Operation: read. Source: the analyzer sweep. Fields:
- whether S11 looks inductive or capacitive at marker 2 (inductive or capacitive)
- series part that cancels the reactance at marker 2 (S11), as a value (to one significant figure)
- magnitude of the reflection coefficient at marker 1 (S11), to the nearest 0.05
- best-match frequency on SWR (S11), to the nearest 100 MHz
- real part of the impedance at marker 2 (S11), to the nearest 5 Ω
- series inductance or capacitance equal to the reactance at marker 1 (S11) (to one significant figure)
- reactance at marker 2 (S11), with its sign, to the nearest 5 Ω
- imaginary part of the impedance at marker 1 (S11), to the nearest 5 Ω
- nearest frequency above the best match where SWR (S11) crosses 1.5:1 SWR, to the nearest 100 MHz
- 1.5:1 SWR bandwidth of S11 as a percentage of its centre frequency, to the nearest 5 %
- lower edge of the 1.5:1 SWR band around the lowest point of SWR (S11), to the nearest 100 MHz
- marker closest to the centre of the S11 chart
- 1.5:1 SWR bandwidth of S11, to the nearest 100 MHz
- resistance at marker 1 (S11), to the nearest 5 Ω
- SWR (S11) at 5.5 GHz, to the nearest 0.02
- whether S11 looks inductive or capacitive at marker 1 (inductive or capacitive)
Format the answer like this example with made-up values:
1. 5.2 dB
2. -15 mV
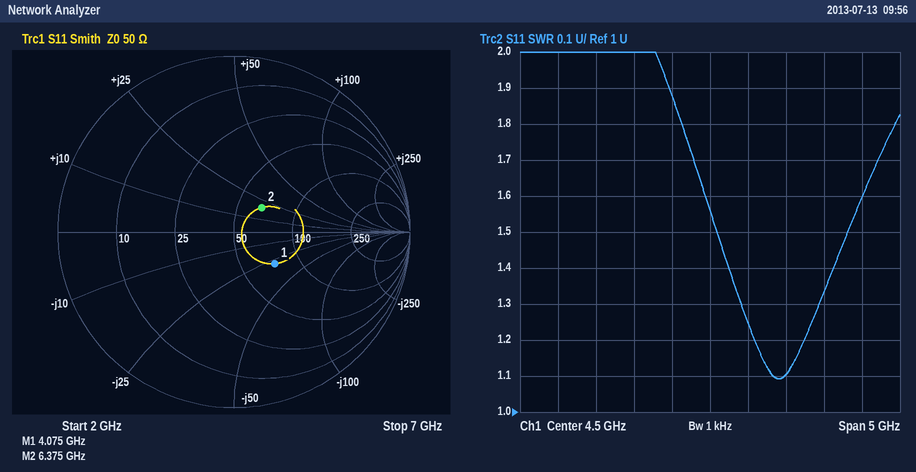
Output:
1. inductive
2. 1 pF
3. 0.30
4. 5.4 GHz
5. 65 Ω
6. 1 pF
7. +20 Ω
8. -30 Ω
9. 6.3 GHz
10. 30 %
11. 4.6 GHz
12. marker 2
13. 1.7 GHz
14. 75 Ω
15. 1.10
16. capacitive
